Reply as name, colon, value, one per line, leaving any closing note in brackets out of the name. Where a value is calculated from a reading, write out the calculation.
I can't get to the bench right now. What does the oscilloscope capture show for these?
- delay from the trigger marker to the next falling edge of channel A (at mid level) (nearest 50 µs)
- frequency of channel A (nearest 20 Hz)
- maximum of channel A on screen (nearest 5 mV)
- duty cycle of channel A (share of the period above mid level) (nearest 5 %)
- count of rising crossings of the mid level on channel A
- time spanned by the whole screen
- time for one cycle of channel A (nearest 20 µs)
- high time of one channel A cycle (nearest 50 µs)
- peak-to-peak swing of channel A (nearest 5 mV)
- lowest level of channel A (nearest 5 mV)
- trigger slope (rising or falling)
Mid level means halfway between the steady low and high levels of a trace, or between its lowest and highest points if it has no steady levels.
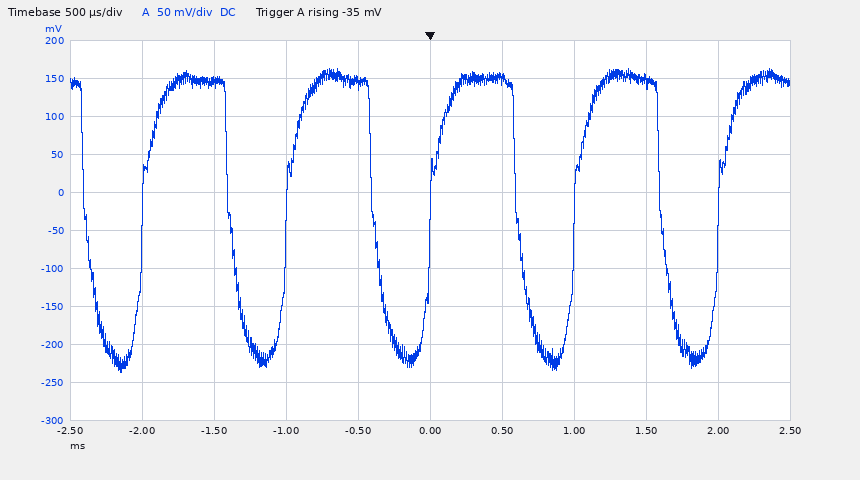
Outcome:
delay from the trigger marker to the next falling edge of channel A (at mid level): 600 µs
frequency of channel A: 1 / 1.00 ms ≈ 1.00 kHz
maximum of channel A on screen: 165 mV
duty cycle of channel A (share of the period above mid level): 600 µs / 1.00 ms ≈ 60 %
count of rising crossings of the mid level on channel A: 5
time spanned by the whole screen: 5 ms
time for one cycle of channel A: 1.00 ms
high time of one channel A cycle: 600 µs
peak-to-peak swing of channel A: 165 mV − (-235 mV) = 400 mV
lowest level of channel A: -235 mV
trigger slope: rising
